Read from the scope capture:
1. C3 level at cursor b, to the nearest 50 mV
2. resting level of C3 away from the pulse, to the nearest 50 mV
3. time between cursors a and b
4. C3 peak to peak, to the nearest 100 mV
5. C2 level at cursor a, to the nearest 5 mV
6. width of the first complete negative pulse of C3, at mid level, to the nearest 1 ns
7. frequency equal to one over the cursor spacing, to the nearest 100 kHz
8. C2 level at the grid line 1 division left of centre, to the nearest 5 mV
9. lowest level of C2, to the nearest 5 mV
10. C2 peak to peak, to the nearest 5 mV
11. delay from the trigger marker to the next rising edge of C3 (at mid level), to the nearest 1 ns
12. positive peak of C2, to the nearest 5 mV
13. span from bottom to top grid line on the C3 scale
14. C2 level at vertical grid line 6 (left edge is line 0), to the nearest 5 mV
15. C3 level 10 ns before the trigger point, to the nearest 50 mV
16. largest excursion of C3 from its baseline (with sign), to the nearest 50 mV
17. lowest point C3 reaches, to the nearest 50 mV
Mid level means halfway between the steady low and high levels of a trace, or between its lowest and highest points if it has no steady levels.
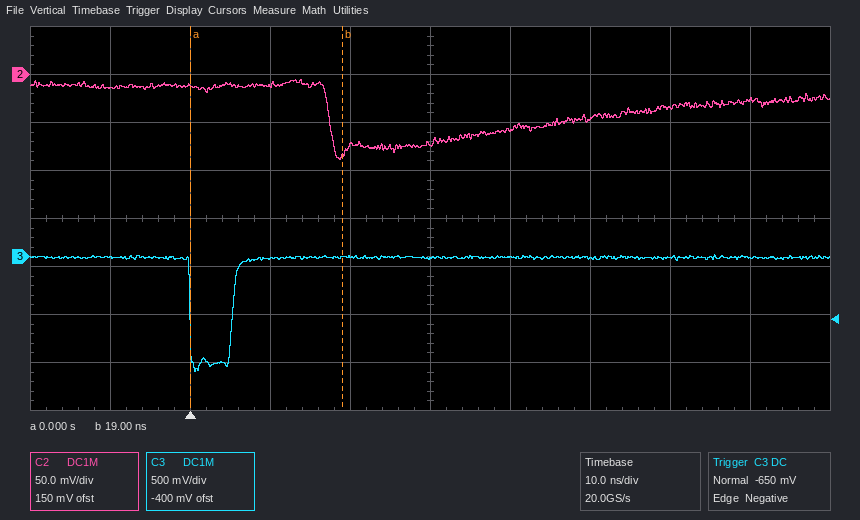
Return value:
0 mV
0 mV
19 ns
1.20 V
-10 mV
5 ns
52.6 MHz
-75 mV
-90 mV
85 mV
5 ns
-5 mV
4 V
-55 mV
0 mV
-1.20 V
-1.20 V
